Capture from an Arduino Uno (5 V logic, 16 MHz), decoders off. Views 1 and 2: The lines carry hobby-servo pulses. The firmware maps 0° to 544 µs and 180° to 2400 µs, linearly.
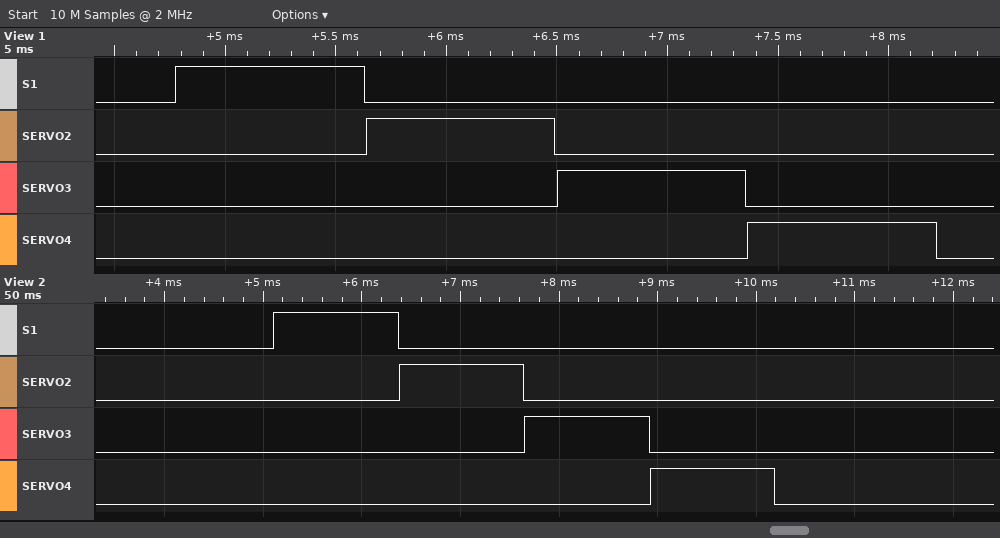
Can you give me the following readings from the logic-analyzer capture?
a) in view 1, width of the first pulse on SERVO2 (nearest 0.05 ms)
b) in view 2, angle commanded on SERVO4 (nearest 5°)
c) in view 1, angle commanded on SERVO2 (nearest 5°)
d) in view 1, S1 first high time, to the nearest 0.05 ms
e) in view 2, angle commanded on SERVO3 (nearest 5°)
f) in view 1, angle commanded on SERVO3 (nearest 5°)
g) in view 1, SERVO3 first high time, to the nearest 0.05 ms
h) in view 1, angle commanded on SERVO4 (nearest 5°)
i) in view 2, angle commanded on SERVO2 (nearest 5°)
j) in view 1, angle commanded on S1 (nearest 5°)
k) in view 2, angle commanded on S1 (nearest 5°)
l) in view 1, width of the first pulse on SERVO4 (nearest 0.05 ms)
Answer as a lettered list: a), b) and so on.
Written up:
a) 0.85 ms
b) 70°
c) 30°
d) 0.85 ms
e) 70°
f) 30°
g) 0.85 ms
h) 30°
i) 70°
j) 30°
k) 70°
l) 0.85 ms
